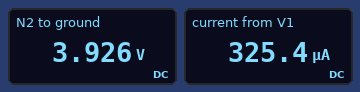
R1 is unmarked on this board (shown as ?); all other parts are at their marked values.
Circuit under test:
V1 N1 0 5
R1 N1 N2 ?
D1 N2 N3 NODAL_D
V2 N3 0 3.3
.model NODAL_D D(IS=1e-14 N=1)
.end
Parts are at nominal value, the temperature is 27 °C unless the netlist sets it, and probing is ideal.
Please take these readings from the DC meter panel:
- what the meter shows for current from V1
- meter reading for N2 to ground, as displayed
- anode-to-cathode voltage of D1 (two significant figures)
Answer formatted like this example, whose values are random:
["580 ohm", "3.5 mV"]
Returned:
["325.4 µA", "3.926 V", "630 mV"]
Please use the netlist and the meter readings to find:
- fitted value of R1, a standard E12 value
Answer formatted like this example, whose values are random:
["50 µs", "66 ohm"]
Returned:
["3.3 kΩ"]
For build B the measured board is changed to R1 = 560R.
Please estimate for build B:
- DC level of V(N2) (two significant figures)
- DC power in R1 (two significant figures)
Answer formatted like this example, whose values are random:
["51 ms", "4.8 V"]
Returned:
["4.0 V", "1.9 mW"]
